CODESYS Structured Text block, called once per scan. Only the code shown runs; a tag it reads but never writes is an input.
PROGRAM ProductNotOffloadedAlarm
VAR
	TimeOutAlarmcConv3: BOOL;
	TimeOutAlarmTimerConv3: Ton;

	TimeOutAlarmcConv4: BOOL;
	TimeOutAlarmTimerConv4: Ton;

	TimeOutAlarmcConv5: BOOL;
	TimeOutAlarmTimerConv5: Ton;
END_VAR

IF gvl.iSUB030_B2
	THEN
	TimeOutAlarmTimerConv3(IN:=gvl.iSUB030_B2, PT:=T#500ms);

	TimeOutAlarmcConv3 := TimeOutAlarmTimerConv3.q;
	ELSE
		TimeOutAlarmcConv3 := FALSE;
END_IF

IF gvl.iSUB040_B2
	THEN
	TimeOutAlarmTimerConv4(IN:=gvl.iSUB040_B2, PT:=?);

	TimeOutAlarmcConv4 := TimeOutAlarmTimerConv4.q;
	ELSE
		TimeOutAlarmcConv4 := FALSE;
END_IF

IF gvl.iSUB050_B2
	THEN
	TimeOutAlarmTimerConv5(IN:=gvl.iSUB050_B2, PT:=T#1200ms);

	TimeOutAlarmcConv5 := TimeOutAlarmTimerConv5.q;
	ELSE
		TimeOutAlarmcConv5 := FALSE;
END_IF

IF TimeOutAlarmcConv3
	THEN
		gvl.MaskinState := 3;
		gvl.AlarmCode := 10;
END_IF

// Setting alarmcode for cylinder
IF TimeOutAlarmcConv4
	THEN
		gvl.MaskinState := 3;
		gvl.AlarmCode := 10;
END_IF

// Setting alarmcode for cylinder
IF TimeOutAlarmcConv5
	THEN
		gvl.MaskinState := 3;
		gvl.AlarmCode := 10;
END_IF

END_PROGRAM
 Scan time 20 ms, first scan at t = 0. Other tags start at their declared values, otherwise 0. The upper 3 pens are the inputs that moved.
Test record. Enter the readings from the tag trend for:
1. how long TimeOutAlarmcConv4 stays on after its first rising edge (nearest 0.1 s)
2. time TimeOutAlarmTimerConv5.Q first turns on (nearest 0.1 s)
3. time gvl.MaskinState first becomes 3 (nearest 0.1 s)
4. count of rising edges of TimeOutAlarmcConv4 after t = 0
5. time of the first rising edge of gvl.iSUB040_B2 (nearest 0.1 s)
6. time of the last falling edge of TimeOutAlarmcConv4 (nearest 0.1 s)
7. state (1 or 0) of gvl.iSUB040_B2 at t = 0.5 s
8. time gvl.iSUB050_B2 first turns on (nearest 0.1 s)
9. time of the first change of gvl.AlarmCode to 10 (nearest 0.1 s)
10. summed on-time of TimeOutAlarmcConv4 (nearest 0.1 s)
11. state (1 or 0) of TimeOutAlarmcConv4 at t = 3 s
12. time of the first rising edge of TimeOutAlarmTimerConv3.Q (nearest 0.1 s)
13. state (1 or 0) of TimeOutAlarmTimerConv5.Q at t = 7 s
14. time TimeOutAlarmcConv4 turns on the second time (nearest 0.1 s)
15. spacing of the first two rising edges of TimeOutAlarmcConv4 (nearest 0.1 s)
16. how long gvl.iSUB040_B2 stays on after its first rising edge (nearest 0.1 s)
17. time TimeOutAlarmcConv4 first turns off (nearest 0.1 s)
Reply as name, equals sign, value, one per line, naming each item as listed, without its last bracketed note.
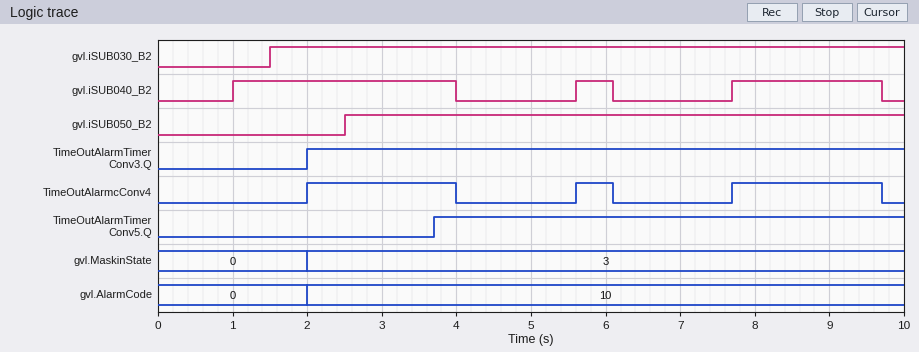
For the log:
how long TimeOutAlarmcConv4 stays on after its first rising edge = 2.0 s
time TimeOutAlarmTimerConv5.Q first turns on = 3.7 s
time gvl.MaskinState first becomes 3 = 2.0 s
count of rising edges of TimeOutAlarmcConv4 after t = 0 = 3
time of the first rising edge of gvl.iSUB040_B2 = 1.0 s
time of the last falling edge of TimeOutAlarmcConv4 = 9.7 s
state (1 or 0) of gvl.iSUB040_B2 at t = 0.5 s = 0
time gvl.iSUB050_B2 first turns on = 2.5 s
time of the first change of gvl.AlarmCode to 10 = 2.0 s
summed on-time of TimeOutAlarmcConv4 = 4.5 s
state (1 or 0) of TimeOutAlarmcConv4 at t = 3 s = 1
time of the first rising edge of TimeOutAlarmTimerConv3.Q = 2.0 s
state (1 or 0) of TimeOutAlarmTimerConv5.Q at t = 7 s = 1
time TimeOutAlarmcConv4 turns on the second time = 5.6 s
spacing of the first two rising edges of TimeOutAlarmcConv4 = 3.6 s
how long gvl.iSUB040_B2 stays on after its first rising edge = 3.0 s
time TimeOutAlarmcConv4 first turns off = 4.0 s
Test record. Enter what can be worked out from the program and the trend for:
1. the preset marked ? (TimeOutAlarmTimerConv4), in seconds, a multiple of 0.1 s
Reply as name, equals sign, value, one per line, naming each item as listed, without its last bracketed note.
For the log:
the preset marked ? (TimeOutAlarmTimerConv4), in seconds, a multiple of 0.1 s = 1.0 s
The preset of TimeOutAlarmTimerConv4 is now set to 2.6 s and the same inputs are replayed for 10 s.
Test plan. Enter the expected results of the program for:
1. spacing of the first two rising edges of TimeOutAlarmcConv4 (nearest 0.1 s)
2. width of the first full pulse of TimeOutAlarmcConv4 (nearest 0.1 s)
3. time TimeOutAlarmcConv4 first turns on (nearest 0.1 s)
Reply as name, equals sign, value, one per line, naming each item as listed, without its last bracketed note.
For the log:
spacing of the first two rising edges of TimeOutAlarmcConv4 = 2.0 s
width of the first full pulse of TimeOutAlarmcConv4 = 0.4 s
time TimeOutAlarmcConv4 first turns on = 3.6 s
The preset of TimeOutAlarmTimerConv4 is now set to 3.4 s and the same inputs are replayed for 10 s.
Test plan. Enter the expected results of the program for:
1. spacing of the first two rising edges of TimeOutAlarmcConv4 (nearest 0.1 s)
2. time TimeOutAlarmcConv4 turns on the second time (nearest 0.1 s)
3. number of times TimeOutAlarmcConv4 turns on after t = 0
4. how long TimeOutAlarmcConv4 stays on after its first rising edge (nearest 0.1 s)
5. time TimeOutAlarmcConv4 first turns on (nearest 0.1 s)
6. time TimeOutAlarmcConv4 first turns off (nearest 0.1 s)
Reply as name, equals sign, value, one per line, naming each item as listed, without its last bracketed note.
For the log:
spacing of the first two rising edges of TimeOutAlarmcConv4 = 2.1 s
time TimeOutAlarmcConv4 turns on the second time = 7.7 s
number of times TimeOutAlarmcConv4 turns on after t = 0 = 2
how long TimeOutAlarmcConv4 stays on after its first rising edge = 0.5 s
time TimeOutAlarmcConv4 first turns on = 5.6 s
time TimeOutAlarmcConv4 first turns off = 6.1 s
